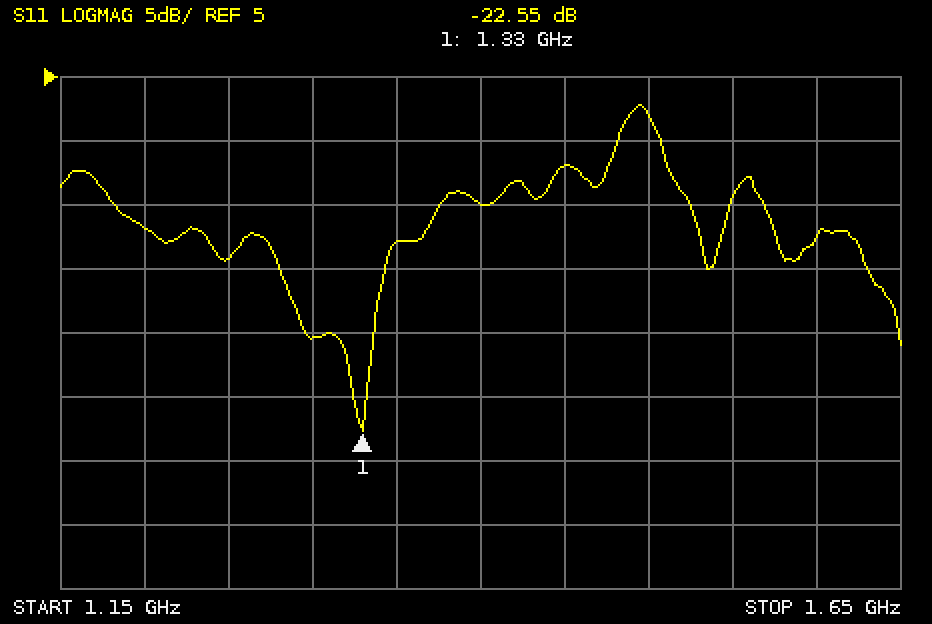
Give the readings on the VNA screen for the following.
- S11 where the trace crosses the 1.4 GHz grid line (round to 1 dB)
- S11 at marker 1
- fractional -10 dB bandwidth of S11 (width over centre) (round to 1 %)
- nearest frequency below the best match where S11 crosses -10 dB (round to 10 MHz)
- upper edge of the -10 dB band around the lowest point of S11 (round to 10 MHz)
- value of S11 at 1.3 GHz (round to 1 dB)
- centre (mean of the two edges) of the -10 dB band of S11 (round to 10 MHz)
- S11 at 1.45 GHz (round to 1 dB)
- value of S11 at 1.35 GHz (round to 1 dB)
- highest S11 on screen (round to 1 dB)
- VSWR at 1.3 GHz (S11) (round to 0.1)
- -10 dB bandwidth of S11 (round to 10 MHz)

-5 dB
-22.55 dB
5 %
1.28 GHz
1.34 GHz
-15 dB
1.31 GHz
-2 dB
-8 dB
3 dB
1.4
60 MHz
